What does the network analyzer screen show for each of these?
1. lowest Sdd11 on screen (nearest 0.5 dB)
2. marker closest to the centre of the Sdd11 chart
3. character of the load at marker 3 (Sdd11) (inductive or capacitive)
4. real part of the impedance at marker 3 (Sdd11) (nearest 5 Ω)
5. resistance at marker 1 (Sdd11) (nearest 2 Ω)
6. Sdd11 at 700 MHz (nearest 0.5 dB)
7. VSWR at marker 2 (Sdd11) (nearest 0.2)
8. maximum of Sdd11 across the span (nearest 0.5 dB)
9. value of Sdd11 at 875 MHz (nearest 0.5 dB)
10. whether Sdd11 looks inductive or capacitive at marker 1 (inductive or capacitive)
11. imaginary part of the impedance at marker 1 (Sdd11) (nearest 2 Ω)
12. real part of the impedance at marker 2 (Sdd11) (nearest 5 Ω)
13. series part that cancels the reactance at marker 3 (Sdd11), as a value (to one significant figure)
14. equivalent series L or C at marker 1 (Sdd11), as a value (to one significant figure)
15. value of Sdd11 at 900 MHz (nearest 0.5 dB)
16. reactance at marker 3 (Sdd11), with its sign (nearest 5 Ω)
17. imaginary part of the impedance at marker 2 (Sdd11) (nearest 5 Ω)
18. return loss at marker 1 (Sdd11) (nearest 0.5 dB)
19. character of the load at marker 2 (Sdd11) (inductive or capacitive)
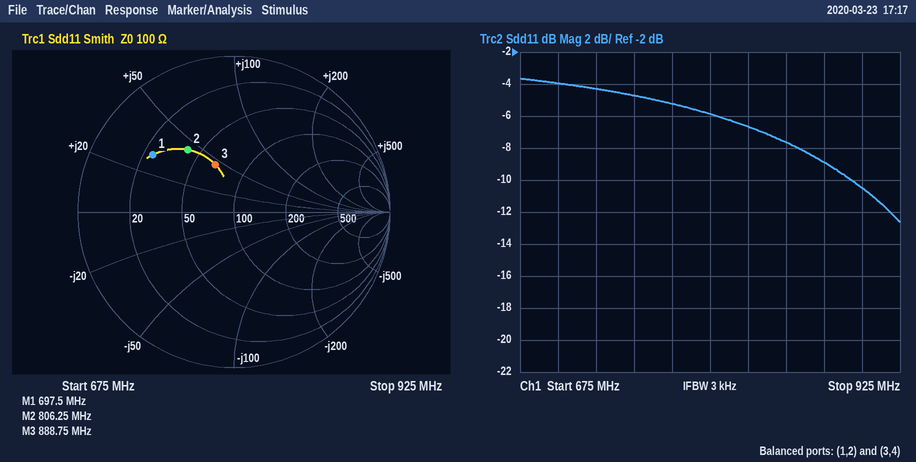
-12.5 dB
marker 3
inductive
65 Ω
24 Ω
-4.0 dB
3.0
-3.5 dB
-9.0 dB
inductive
+30 Ω
40 Ω
4 pF
7 nH
-10.5 dB
+45 Ω
+45 Ω
4.0 dB
inductive
